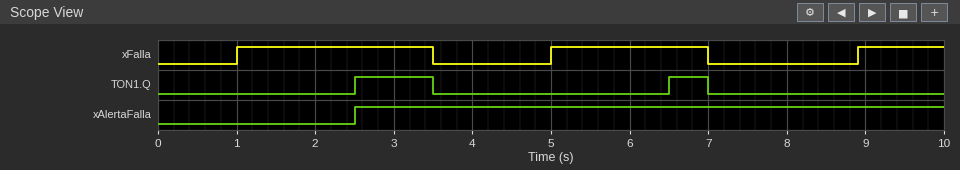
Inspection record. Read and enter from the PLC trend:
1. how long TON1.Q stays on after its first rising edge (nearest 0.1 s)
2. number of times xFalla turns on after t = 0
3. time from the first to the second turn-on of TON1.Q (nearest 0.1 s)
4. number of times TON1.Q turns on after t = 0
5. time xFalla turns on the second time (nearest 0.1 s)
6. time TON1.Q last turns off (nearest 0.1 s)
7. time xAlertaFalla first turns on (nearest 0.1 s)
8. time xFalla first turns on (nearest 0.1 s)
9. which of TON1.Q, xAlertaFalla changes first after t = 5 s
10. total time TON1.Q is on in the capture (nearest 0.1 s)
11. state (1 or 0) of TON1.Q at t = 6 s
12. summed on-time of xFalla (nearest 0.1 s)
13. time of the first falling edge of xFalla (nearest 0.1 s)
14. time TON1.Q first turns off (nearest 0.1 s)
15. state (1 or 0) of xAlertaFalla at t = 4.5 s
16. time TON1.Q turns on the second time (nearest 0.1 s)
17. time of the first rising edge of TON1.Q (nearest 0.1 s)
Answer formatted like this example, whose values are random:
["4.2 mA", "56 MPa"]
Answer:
["1.0 s", "3", "4.0 s", "2", "5.0 s", "7.0 s", "2.5 s", "1.0 s", "TON1.Q", "1.5 s", "0", "5.6 s", "3.5 s", "3.5 s", "1", "6.5 s", "2.5 s"]
